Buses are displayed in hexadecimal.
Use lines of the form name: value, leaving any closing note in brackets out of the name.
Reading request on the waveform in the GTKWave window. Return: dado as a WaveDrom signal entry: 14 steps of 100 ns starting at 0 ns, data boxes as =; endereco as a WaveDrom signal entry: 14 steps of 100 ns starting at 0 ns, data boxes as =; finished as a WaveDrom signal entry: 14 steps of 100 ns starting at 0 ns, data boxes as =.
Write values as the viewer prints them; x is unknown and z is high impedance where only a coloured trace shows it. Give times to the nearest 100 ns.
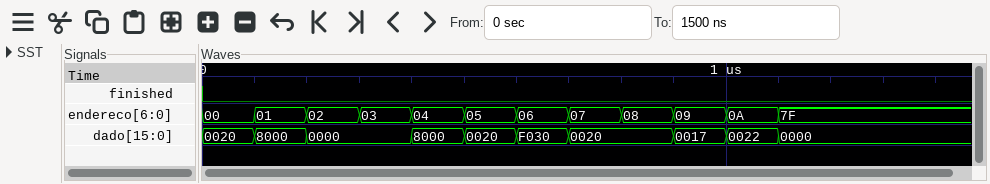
dado as a WaveDrom signal entry: 14 steps of 100 ns starting at 0 ns, data boxes as =: {name: 'dado', wave: '===.====.===..', data: '0020 8000 0000 8000 0020 F030 0020 0017 0022 0000'}
endereco as a WaveDrom signal entry: 14 steps of 100 ns starting at 0 ns, data boxes as =: {name: 'endereco', wave: '============..', data: '00 01 02 03 04 05 06 07 08 09 0A 7F'}
finished as a WaveDrom signal entry: 14 steps of 100 ns starting at 0 ns, data boxes as =: {name: 'finished', wave: '0.............'}
